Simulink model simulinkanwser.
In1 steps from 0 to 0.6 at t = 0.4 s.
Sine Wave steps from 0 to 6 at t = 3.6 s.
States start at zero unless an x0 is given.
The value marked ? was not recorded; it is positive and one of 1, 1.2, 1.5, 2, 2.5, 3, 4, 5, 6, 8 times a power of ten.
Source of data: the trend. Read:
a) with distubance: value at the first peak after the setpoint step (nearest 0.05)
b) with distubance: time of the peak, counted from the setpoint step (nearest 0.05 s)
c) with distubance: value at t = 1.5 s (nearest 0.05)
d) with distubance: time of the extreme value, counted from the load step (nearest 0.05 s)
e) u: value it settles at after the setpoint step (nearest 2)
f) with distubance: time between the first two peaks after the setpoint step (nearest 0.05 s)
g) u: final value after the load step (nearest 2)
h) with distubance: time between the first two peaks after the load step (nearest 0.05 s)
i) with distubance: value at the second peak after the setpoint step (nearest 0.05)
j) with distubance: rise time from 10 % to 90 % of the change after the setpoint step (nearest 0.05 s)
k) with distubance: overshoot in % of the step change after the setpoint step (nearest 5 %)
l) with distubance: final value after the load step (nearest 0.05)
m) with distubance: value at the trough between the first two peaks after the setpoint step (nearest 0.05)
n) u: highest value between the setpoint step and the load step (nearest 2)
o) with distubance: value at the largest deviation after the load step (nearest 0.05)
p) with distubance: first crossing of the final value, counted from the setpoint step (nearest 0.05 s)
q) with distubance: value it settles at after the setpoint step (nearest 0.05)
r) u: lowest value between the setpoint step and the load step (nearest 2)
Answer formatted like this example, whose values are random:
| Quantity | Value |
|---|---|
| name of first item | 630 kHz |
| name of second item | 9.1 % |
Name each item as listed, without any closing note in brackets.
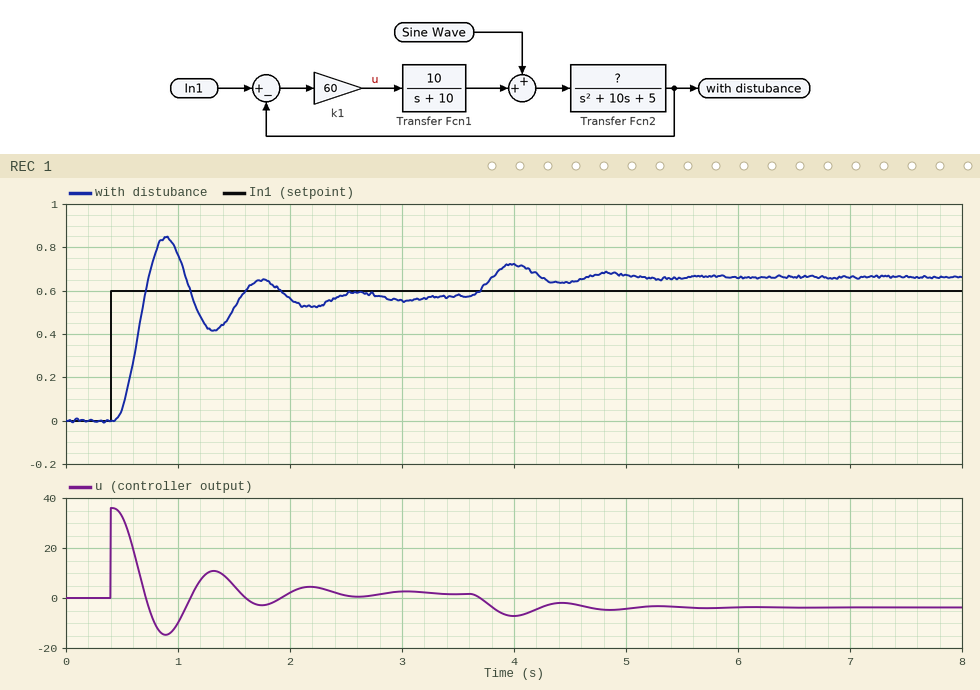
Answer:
| Quantity | Value |
|---|---|
| with distubance: value at the first peak after the setpoint step | 0.85 |
| with distubance: time of the peak, counted from the setpoint step | 0.50 s |
| with distubance: value at t = 1.5 s | 0.50 |
| with distubance: time of the extreme value, counted from the load step | 0.40 s |
| u: value it settles at after the setpoint step | 2 |
| with distubance: time between the first two peaks after the setpoint step | 0.85 s |
| u: final value after the load step | -4 |
| with distubance: time between the first two peaks after the load step | 0.85 s |
| with distubance: value at the second peak after the setpoint step | 0.65 |
| with distubance: rise time from 10 % to 90 % of the change after the setpoint step | 0.20 s |
| with distubance: overshoot in % of the step change after the setpoint step | 50 % |
| with distubance: final value after the load step | 0.65 |
| with distubance: value at the trough between the first two peaks after the setpoint step | 0.40 |
| u: highest value between the setpoint step and the load step | 36 |
| with distubance: value at the largest deviation after the load step | 0.70 |
| with distubance: first crossing of the final value, counted from the setpoint step | 0.30 s |
| with distubance: value it settles at after the setpoint step | 0.55 |
| u: lowest value between the setpoint step and the load step | -14 |
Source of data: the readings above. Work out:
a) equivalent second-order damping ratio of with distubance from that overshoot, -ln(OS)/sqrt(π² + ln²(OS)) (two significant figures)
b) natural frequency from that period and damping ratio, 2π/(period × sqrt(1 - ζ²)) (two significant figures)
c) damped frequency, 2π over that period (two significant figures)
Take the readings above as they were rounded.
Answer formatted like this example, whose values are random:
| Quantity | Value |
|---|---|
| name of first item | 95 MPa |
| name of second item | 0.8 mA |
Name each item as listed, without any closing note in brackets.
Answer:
| Quantity | Value |
|---|---|
| equivalent second-order damping ratio of with distubance from that overshoot, -ln(OS)/sqrt(π² + ln²(OS)) | 0.22 |
| natural frequency from that period and damping ratio, 2π/(period × sqrt(1 - ζ²)) | 7.6 rad/s |
| damped frequency, 2π over that period | 7.4 rad/s |
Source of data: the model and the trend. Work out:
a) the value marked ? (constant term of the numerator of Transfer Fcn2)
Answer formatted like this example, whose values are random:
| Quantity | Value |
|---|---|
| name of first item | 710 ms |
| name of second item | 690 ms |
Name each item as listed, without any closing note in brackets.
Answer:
| Quantity | Value |
|---|---|
| the value marked ? | 1.5 |
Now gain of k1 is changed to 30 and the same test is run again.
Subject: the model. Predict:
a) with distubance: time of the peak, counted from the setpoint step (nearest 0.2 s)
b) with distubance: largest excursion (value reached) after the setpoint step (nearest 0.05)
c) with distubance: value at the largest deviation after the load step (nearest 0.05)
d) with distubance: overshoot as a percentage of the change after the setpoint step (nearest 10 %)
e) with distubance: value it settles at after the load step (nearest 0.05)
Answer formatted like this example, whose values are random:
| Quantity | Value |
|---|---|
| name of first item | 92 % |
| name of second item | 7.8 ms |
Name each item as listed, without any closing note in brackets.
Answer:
| Quantity | Value |
|---|---|
| with distubance: time of the peak, counted from the setpoint step | 0.6 s |
| with distubance: largest excursion (value reached) after the setpoint step | 0.65 |
| with distubance: value at the largest deviation after the load step | 0.75 |
| with distubance: overshoot as a percentage of the change after the setpoint step | 20 % |
| with distubance: value it settles at after the load step | 0.70 |
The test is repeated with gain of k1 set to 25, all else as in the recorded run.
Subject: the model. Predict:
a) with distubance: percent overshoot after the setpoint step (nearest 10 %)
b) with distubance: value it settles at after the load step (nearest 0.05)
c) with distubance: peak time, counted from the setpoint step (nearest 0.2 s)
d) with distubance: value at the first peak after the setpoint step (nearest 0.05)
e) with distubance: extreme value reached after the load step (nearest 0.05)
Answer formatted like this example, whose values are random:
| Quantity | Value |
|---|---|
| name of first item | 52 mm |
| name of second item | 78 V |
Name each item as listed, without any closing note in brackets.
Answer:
| Quantity | Value |
|---|---|
| with distubance: percent overshoot after the setpoint step | 20 % |
| with distubance: value it settles at after the load step | 0.75 |
| with distubance: peak time, counted from the setpoint step | 0.8 s |
| with distubance: value at the first peak after the setpoint step | 0.60 |
| with distubance: extreme value reached after the load step | 0.80 |
